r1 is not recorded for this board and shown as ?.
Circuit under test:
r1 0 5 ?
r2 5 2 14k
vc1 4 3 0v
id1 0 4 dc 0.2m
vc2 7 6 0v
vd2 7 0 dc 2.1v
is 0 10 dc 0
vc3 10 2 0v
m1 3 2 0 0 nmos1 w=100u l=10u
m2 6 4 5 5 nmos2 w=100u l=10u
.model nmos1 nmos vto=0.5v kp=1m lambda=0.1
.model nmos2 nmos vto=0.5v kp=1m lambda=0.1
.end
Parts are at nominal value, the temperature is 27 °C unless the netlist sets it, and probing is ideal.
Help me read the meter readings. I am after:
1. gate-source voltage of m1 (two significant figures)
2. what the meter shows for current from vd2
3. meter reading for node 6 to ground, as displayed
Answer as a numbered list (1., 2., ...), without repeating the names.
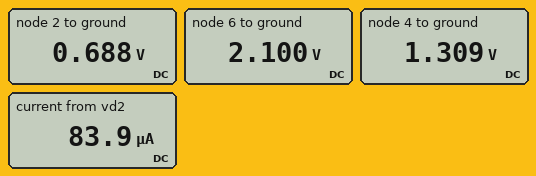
1. 690 mV
2. 83.9 µA
3. 2.100 V
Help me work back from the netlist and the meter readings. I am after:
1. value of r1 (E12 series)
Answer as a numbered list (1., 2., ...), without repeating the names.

1. 8.2 kΩ
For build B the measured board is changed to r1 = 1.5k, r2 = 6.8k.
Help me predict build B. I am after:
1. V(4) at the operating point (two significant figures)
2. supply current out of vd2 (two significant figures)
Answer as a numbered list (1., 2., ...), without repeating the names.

1. 1.5 V
2. 460 µA
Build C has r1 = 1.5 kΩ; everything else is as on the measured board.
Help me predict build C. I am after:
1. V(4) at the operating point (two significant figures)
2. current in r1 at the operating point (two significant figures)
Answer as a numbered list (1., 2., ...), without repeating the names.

1. 1.5 V
2. 460 µA
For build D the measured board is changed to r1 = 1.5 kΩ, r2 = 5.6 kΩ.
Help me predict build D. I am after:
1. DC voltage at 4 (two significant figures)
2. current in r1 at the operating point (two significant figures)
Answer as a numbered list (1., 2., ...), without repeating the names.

1. 1.5 V
2. 460 µA
